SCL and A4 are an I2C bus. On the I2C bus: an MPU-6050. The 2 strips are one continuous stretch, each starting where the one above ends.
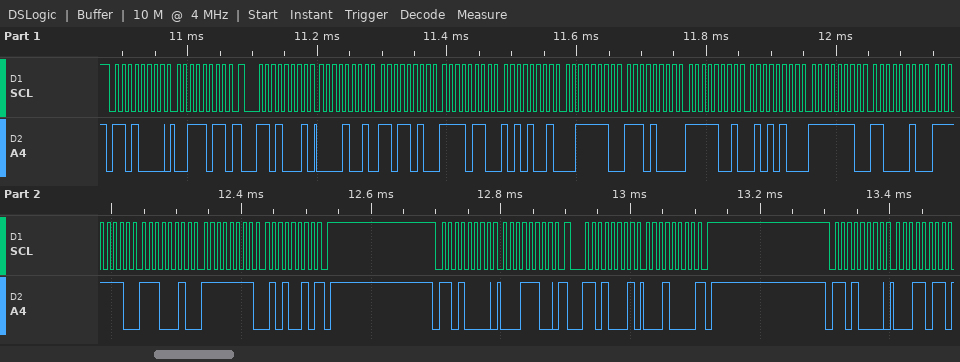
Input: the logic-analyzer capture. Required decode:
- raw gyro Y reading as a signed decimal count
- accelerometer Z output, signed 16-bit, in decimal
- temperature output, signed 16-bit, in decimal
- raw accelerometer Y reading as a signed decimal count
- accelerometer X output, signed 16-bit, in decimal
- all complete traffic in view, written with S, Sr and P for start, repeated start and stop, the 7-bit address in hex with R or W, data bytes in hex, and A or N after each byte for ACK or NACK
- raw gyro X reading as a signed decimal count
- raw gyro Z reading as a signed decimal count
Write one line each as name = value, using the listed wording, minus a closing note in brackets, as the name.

raw gyro Y reading as a signed decimal count = -286
accelerometer Z output, signed 16-bit, in decimal = 16104
temperature output, signed 16-bit, in decimal = -1708
raw accelerometer Y reading as a signed decimal count = -2391
accelerometer X output, signed 16-bit, in decimal = 2522
all complete traffic in view, written with S, Sr and P for start, repeated start and stop, the 7-bit address in hex with R or W, data bytes in hex, and A or N after each byte for ACK or NACK = S 68W A 3B A Sr 68R A 09 A DA A F6 A A9 A 3E A E8 A F9 A 54 A FE A C2 A FE A E2 A FF A 52 N P S 68W A 1C A Sr 68R A 10 N P S 68W A 1B A
raw gyro X reading as a signed decimal count = -318
raw gyro Z reading as a signed decimal count = -174
